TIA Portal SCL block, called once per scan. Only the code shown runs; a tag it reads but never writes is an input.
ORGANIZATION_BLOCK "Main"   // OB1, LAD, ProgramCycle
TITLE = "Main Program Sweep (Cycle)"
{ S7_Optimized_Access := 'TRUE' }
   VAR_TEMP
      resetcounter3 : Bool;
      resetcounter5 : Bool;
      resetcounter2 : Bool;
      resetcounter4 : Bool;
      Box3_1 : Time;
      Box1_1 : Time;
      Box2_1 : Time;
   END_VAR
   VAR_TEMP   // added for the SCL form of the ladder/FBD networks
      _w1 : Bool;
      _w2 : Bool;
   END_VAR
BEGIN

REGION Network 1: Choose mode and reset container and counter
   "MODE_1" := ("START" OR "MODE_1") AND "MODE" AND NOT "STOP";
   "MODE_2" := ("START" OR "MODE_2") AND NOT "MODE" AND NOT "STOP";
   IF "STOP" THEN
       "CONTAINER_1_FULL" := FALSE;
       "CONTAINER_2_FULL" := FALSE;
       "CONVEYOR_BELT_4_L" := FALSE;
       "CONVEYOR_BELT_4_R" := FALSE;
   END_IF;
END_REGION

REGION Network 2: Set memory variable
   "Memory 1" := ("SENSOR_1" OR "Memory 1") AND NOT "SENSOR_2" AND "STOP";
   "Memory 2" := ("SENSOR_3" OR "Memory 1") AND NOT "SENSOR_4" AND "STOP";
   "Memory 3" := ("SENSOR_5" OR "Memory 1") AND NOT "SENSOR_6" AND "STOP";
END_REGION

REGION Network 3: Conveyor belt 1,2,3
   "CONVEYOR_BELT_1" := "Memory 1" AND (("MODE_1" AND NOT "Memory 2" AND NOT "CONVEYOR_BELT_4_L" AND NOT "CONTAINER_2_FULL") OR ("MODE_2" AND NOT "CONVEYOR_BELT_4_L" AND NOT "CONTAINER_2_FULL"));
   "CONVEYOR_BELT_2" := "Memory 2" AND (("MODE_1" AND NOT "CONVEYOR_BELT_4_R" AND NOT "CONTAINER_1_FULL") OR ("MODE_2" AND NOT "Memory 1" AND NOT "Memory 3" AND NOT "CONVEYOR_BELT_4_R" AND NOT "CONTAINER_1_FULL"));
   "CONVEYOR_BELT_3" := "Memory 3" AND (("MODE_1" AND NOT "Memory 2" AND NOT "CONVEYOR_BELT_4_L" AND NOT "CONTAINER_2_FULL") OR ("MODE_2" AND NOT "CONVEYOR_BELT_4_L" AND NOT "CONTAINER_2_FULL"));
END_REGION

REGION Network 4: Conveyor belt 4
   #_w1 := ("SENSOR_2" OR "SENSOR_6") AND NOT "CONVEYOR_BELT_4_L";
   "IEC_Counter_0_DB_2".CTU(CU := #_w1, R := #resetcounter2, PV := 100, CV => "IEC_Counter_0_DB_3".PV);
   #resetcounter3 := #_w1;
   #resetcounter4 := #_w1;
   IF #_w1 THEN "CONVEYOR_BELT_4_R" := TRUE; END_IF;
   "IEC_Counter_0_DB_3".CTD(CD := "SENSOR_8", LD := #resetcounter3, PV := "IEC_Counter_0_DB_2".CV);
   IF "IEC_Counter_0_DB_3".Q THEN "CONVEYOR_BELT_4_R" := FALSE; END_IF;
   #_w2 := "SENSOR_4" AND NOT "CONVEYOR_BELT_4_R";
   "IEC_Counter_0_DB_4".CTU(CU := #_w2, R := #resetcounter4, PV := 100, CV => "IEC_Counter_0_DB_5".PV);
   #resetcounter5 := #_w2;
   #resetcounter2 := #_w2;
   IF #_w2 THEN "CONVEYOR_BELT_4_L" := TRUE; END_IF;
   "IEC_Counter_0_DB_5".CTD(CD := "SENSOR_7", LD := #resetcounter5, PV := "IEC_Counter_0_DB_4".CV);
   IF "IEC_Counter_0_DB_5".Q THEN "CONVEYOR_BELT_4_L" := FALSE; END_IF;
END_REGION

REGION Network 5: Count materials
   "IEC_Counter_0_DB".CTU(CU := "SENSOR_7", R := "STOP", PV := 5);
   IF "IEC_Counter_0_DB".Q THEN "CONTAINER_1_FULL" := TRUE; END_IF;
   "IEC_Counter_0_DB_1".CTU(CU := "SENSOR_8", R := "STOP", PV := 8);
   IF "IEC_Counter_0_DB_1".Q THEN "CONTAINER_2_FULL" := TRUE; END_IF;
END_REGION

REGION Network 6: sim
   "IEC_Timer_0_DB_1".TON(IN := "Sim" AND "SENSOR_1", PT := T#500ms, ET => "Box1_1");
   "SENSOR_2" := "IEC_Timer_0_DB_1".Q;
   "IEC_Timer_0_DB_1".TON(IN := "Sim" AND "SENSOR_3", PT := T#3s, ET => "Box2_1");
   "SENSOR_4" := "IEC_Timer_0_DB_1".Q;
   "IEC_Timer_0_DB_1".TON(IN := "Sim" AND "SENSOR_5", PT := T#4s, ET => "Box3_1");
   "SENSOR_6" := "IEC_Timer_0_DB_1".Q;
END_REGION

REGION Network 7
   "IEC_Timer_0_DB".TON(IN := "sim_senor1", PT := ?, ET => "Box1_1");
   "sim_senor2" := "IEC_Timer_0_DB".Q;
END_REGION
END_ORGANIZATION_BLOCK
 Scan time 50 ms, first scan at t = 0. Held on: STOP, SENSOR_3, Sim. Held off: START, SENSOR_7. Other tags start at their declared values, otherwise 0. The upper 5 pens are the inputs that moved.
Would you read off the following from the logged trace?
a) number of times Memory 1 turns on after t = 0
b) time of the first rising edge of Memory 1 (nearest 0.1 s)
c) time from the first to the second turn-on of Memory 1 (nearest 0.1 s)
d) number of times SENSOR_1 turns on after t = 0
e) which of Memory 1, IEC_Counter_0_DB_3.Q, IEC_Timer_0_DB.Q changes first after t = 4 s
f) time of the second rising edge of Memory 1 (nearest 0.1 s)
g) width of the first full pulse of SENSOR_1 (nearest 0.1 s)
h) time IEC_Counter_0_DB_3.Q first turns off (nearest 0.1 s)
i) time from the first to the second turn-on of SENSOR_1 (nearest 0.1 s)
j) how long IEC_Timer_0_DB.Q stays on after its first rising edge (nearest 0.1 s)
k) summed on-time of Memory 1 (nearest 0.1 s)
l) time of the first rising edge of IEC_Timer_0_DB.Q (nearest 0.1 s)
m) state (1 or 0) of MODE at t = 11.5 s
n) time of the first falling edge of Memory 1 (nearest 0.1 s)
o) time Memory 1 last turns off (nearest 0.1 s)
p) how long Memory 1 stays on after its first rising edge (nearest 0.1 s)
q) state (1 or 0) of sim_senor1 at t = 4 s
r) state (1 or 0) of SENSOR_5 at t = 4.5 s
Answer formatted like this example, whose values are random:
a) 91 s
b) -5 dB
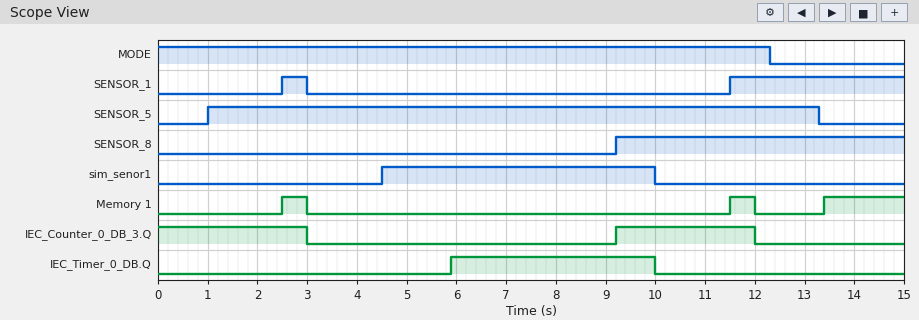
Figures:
a) 3
b) 2.5 s
c) 9.0 s
d) 2
e) IEC_Timer_0_DB.Q
f) 11.5 s
g) 0.5 s
h) 3.0 s
i) 9.0 s
j) 4.1 s
k) 2.6 s
l) 5.9 s
m) 1
n) 3.0 s
o) 12.0 s
p) 0.5 s
q) 0
r) 1
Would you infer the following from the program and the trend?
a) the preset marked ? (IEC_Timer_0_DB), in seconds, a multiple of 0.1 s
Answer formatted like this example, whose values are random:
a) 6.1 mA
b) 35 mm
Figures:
a) 1.4 s
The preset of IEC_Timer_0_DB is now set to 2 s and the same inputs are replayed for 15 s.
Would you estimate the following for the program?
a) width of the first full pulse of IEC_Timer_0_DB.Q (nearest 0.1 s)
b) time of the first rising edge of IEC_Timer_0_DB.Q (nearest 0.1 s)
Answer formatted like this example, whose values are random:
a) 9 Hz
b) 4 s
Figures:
a) 3.5 s
b) 6.5 s
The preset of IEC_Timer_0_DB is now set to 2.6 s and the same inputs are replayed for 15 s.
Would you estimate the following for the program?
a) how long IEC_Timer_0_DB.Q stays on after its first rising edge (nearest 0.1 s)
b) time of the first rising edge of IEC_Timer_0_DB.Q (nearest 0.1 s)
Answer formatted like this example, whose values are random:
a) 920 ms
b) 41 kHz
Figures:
a) 2.9 s
b) 7.1 s
